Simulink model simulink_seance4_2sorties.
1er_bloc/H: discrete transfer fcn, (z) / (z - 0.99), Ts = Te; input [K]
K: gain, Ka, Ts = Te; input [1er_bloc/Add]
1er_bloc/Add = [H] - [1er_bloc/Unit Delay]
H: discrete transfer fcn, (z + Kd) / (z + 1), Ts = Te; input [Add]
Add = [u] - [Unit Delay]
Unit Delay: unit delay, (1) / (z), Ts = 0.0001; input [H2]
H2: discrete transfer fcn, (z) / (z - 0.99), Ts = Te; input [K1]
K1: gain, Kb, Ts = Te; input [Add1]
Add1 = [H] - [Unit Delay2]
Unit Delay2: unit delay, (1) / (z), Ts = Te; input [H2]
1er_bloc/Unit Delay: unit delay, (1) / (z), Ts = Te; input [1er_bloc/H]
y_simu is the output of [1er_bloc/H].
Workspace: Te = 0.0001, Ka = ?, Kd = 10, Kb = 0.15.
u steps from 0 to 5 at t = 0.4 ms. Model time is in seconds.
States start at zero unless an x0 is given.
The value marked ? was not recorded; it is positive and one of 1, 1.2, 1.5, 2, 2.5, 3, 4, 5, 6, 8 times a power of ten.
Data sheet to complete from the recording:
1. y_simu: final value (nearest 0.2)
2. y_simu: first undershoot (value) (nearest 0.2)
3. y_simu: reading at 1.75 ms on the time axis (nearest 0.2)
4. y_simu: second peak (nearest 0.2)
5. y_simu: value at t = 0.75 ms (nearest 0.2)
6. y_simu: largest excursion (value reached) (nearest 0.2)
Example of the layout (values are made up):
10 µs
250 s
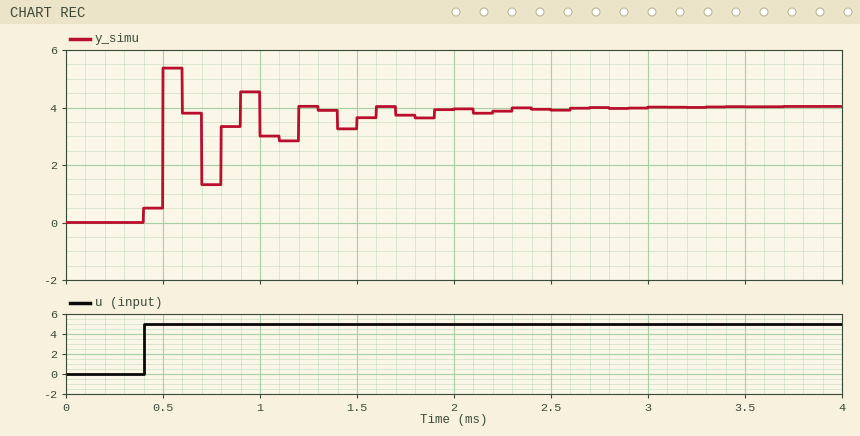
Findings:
4.0
1.4
3.8
4.6
1.4
5.4
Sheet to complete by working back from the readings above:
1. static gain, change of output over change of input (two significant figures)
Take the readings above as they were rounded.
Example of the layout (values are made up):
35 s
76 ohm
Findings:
0.80
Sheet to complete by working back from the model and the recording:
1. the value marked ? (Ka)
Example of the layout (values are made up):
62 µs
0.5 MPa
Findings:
0.1
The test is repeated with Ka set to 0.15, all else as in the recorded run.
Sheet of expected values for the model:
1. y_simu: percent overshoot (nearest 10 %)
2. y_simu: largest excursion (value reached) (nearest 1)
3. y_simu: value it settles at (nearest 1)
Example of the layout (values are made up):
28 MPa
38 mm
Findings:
90 %
8
4
